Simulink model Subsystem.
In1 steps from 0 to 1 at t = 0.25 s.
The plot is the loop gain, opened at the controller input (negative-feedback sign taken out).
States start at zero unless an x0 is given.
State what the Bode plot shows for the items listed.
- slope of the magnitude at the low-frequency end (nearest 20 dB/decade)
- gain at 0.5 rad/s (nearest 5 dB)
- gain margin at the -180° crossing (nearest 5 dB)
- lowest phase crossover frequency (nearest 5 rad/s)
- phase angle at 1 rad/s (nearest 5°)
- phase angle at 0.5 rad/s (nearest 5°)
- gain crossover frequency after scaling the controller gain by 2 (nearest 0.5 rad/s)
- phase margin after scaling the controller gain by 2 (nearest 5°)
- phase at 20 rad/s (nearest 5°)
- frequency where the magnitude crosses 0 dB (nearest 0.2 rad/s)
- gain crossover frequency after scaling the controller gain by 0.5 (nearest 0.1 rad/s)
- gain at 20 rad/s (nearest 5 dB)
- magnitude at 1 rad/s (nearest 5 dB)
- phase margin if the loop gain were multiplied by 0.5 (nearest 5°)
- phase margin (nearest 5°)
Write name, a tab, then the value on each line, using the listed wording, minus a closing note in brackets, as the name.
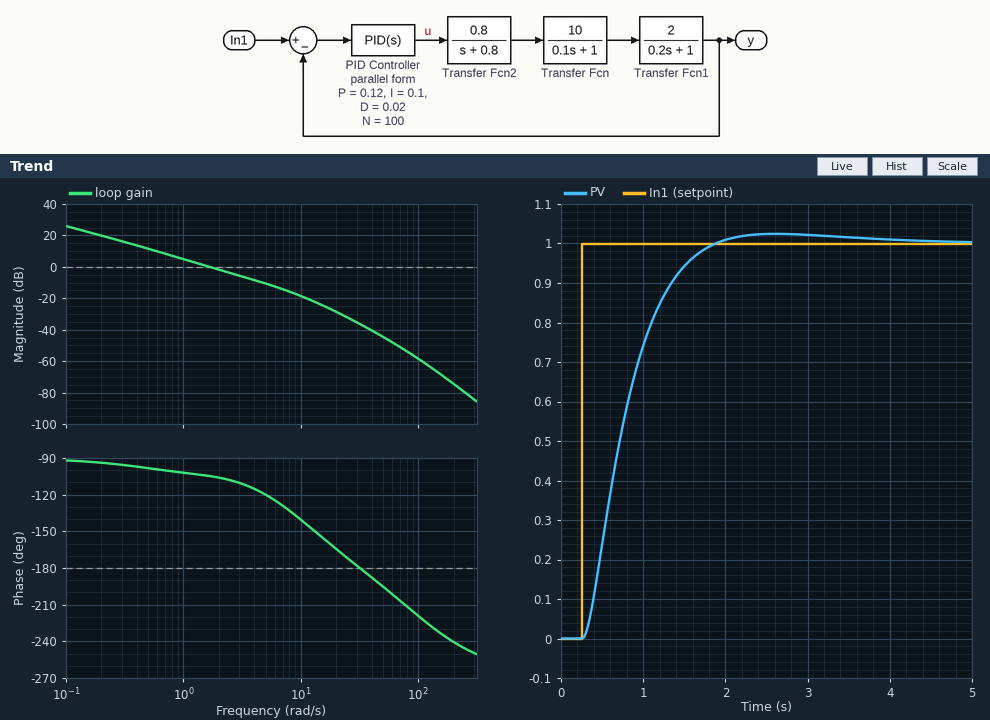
slope of the magnitude at the low-frequency end	-20 dB/decade
gain at 0.5 rad/s	10 dB
gain margin at the -180° crossing	35 dB
lowest phase crossover frequency	30 rad/s
phase angle at 1 rad/s	-100°
phase angle at 0.5 rad/s	-100°
gain crossover frequency after scaling the controller gain by 2	3.0 rad/s
phase margin after scaling the controller gain by 2	70°
phase at 20 rad/s	-165°
frequency where the magnitude crosses 0 dB	1.6 rad/s
gain crossover frequency after scaling the controller gain by 0.5	0.9 rad/s
gain at 20 rad/s	-30 dB
magnitude at 1 rad/s	5 dB
phase margin if the loop gain were multiplied by 0.5	80°
phase margin	75°
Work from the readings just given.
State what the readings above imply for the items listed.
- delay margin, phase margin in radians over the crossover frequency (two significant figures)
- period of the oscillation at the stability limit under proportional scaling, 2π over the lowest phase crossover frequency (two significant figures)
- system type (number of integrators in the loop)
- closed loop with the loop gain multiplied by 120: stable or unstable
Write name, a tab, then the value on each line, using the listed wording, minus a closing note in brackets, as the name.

delay margin, phase margin in radians over the crossover frequency	0.82 s
period of the oscillation at the stability limit under proportional scaling, 2π over the lowest phase crossover frequency	0.21 s
system type	1
closed loop with the loop gain multiplied by 120: stable or unstable	unstable
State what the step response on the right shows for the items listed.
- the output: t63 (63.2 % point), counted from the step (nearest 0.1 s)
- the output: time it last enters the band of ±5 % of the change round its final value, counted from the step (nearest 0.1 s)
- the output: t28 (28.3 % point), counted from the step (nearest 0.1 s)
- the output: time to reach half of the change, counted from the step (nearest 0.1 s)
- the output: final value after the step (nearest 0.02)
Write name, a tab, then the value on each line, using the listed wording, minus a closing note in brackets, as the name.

the output: t63 (63.2 % point), counted from the step	0.6 s
the output: time it last enters the band of ±5 % of the change round its final value, counted from the step	1.3 s
the output: t28 (28.3 % point), counted from the step	0.3 s
the output: time to reach half of the change, counted from the step	0.5 s
the output: final value after the step	1.00
